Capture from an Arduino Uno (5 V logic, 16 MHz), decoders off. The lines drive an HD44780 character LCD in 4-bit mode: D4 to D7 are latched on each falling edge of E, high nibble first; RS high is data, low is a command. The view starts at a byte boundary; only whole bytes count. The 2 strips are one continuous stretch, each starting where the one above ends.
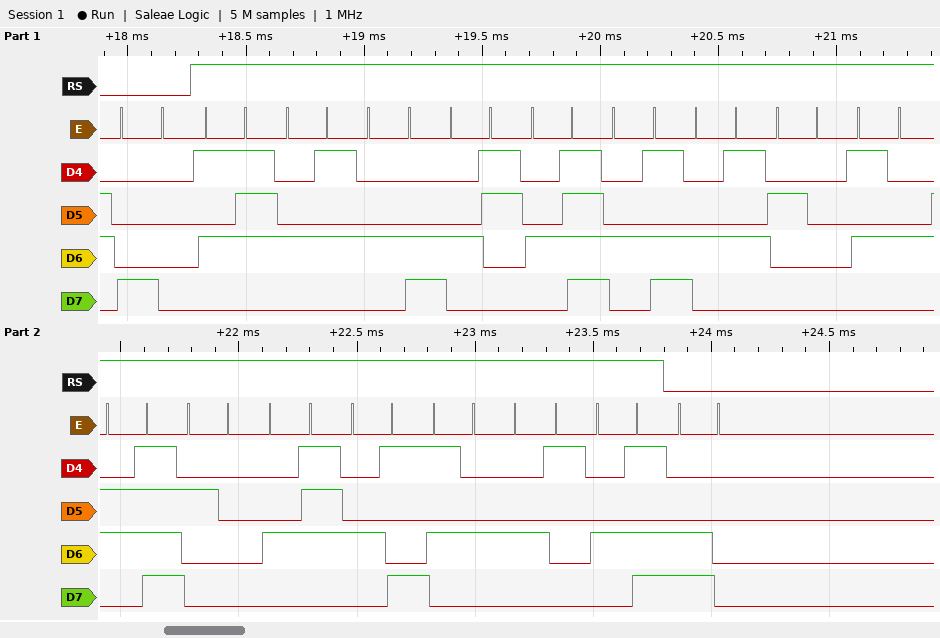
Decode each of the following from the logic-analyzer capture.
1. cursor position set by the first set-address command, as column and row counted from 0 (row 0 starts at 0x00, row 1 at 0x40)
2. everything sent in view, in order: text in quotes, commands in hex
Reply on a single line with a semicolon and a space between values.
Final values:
column 0, row 0; 0x80 "WELCOME To GITAM" 0xC0
